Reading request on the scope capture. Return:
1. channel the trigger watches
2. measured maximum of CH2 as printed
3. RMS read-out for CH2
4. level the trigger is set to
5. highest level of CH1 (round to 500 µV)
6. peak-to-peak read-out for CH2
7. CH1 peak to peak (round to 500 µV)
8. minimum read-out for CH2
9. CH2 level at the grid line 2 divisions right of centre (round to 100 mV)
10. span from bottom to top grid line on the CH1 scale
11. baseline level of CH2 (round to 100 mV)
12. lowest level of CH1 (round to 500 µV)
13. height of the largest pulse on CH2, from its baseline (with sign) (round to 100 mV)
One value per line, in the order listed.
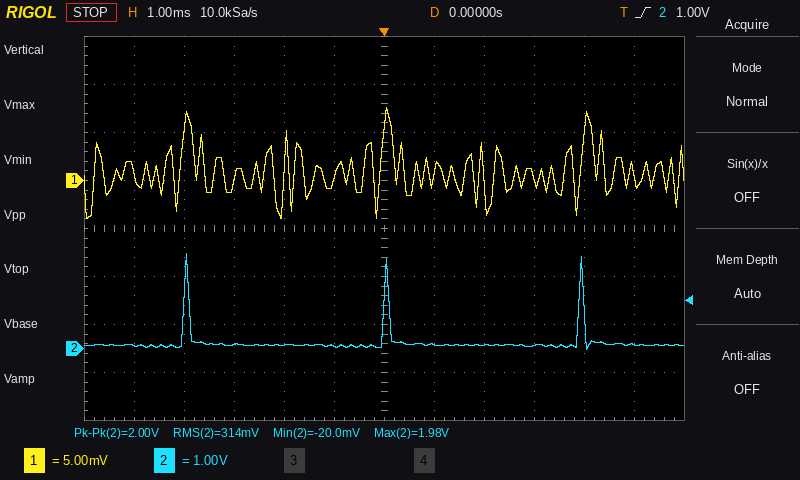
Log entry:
CH2
1.98 V
314 mV
1.00 V
7.5 mV
2.00 V
11.5 mV
-20.0 mV
100 mV
40 mV
100 mV
-4.0 mV
+1.9 V
